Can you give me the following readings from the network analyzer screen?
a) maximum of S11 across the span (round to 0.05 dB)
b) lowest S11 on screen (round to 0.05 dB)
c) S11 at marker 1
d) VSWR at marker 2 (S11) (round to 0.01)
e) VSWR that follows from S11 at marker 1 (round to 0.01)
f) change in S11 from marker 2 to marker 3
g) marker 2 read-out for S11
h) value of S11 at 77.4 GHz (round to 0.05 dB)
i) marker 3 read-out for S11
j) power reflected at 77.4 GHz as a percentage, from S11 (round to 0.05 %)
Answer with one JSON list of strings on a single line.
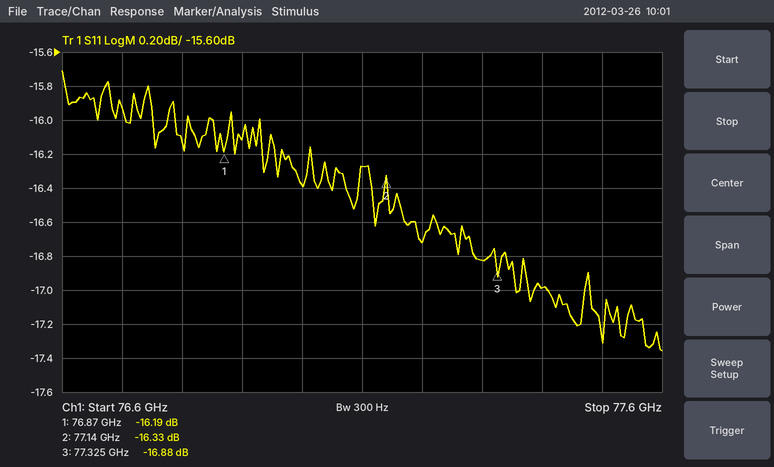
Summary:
["-15.70 dB", "-17.35 dB", "-16.19 dB", "1.36", "1.37", "-0.55 dB", "-16.33 dB", "-17.00 dB", "-16.88 dB", "2.00 %"]
